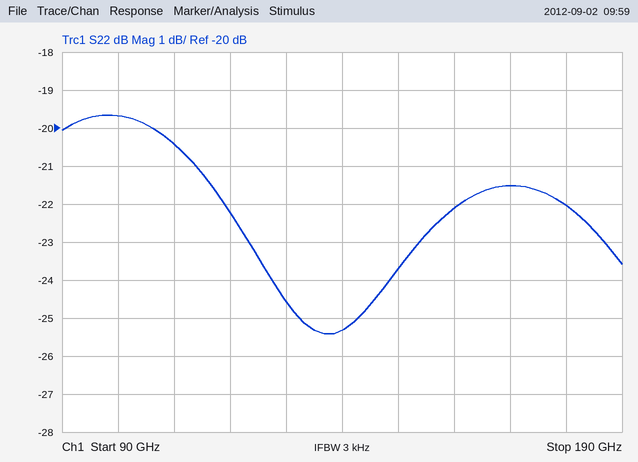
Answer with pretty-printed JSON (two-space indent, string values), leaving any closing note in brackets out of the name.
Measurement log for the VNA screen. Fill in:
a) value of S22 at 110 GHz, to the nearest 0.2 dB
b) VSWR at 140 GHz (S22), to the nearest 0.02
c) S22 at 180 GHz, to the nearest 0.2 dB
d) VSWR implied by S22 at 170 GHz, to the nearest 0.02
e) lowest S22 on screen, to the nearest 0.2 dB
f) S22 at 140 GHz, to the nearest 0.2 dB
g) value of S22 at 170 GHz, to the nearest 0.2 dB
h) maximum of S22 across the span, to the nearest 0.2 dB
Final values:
{
  "value of S22 at 110 GHz, to the nearest 0.2 dB": "-20.4 dB",
  "VSWR at 140 GHz (S22), to the nearest 0.02": "1.12",
  "S22 at 180 GHz, to the nearest 0.2 dB": "-22.0 dB",
  "VSWR implied by S22 at 170 GHz, to the nearest 0.02": "1.18",
  "lowest S22 on screen, to the nearest 0.2 dB": "-25.4 dB",
  "S22 at 140 GHz, to the nearest 0.2 dB": "-25.4 dB",
  "value of S22 at 170 GHz, to the nearest 0.2 dB": "-21.6 dB",
  "maximum of S22 across the span, to the nearest 0.2 dB": "-19.6 dB"
}
